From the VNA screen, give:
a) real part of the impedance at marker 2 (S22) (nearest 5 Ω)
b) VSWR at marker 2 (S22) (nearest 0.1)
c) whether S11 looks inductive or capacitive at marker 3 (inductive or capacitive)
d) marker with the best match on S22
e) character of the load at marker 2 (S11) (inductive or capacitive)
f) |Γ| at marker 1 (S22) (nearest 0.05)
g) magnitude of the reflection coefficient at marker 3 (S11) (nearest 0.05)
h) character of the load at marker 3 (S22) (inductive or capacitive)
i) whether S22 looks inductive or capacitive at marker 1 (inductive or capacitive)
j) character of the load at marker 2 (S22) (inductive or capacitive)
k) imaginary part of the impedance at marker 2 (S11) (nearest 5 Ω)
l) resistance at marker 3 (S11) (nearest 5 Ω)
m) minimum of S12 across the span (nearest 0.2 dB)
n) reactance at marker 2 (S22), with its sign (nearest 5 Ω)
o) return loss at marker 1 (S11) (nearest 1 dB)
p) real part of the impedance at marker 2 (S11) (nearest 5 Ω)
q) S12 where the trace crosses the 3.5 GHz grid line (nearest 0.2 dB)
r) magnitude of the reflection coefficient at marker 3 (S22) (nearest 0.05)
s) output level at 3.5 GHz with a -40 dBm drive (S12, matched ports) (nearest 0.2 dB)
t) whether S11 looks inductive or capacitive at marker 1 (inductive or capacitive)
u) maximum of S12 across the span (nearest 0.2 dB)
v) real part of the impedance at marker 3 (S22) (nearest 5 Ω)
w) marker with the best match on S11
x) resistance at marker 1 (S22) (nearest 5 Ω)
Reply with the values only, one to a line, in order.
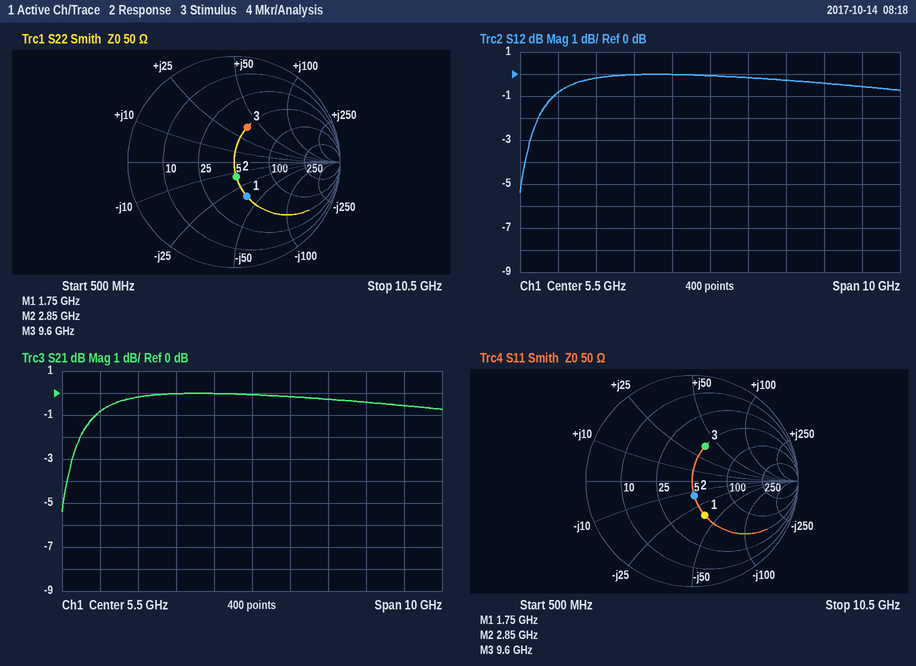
50 Ω
1.3
inductive
marker 2
capacitive
0.35
0.35
inductive
capacitive
capacitive
-15 Ω
50 Ω
-5.4 dB
-15 Ω
9 dB
50 Ω
0.0 dB
0.35
-40.0 dBm
capacitive
0.0 dB
50 Ω
marker 2
50 Ω
